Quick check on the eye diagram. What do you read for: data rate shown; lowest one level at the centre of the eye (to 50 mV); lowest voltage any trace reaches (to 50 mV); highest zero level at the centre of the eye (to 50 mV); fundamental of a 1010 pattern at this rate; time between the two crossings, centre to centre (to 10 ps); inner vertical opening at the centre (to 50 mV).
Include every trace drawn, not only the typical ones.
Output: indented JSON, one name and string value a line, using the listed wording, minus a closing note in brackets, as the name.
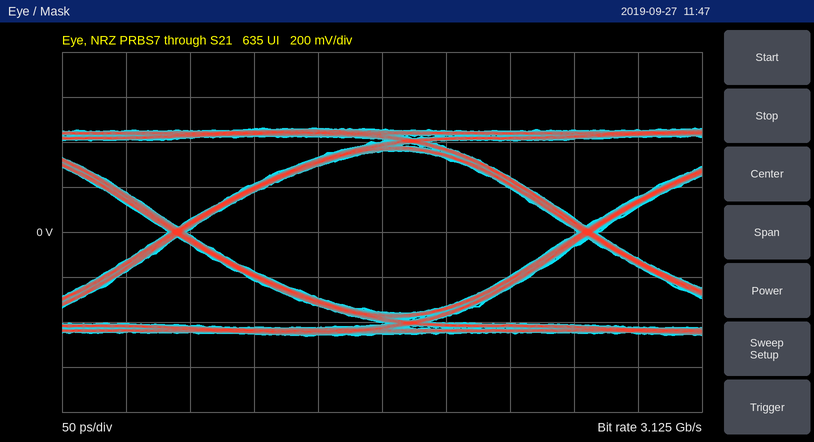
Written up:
{
  "data rate shown": "3.125 Gb/s",
  "lowest one level at the centre of the eye": "350 mV",
  "lowest voltage any trace reaches": "-450 mV",
  "highest zero level at the centre of the eye": "-350 mV",
  "fundamental of a 1010 pattern at this rate": "1.5625 GHz",
  "time between the two crossings, centre to centre": "320 ps",
  "inner vertical opening at the centre": "700 mV"
}
